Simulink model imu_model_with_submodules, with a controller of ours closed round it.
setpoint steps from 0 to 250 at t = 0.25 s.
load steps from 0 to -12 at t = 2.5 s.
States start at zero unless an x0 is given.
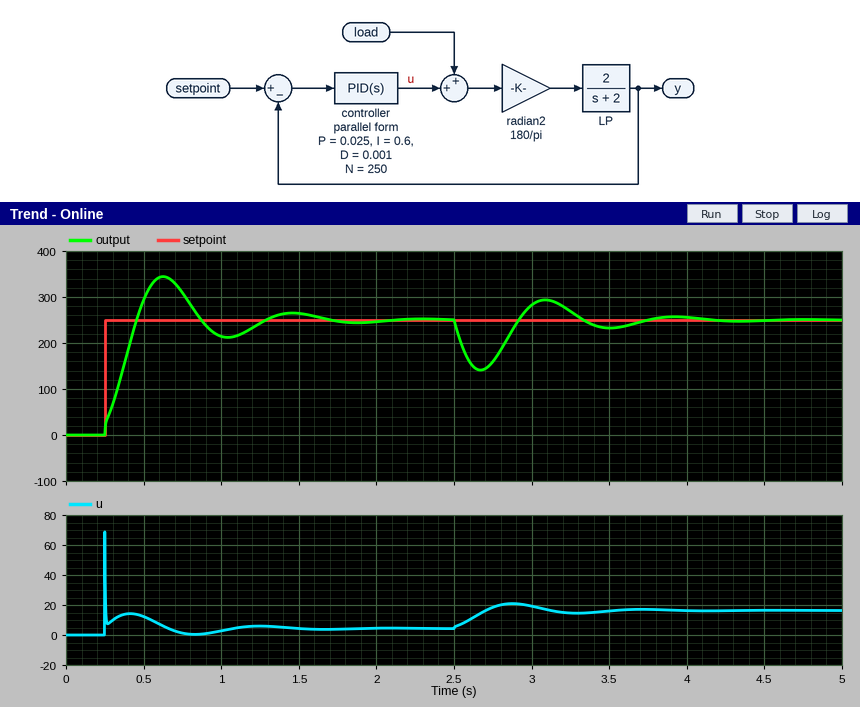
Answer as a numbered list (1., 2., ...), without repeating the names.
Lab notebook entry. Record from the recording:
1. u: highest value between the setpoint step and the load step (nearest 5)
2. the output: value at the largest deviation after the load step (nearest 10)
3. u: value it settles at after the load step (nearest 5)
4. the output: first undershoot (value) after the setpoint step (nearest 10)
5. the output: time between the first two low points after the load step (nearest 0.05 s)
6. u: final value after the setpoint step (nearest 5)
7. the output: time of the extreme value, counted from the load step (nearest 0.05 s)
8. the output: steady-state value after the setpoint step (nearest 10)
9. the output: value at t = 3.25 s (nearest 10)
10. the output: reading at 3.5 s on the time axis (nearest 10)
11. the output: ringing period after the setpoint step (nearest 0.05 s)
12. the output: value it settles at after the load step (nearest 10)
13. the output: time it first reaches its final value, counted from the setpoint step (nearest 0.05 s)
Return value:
1. 70
2. 140
3. 15
4. 210
5. 0.85 s
6. 5
7. 0.15 s
8. 250
9. 270
10. 230
11. 0.85 s
12. 250
13. 0.20 s
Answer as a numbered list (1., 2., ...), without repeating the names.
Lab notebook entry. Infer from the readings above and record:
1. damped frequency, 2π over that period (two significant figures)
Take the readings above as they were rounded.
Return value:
1. 7.4 rad/s
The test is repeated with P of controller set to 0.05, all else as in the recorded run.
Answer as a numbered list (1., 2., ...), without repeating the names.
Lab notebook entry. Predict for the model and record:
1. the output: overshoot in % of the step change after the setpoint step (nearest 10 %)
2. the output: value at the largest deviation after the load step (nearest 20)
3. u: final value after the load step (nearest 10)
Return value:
1. 20 %
2. 160
3. 20
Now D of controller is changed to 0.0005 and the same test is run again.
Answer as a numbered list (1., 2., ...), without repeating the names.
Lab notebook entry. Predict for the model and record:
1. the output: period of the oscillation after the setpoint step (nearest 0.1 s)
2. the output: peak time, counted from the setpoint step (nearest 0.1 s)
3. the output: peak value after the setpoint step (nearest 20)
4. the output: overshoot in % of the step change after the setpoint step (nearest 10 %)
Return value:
1. 0.8 s
2. 0.4 s
3. 340
4. 40 %
